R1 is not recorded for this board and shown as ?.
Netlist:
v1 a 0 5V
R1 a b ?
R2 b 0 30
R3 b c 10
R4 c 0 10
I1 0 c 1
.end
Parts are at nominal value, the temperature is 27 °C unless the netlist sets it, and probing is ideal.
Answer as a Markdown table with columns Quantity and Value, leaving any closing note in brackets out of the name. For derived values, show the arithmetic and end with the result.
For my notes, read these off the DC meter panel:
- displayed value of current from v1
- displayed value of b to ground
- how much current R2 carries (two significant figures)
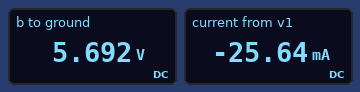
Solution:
| Quantity | Value |
|---|---|
| displayed value of current from v1 | -25.64 mA |
| displayed value of b to ground | 5.692 V |
| how much current R2 carries | (5.692 V) / 30 Ω = 190 mA |
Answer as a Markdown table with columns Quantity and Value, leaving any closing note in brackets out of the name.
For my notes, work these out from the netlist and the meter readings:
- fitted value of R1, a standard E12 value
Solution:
| Quantity | Value |
|---|---|
| fitted value of R1, a standard E12 value | 27 Ω |
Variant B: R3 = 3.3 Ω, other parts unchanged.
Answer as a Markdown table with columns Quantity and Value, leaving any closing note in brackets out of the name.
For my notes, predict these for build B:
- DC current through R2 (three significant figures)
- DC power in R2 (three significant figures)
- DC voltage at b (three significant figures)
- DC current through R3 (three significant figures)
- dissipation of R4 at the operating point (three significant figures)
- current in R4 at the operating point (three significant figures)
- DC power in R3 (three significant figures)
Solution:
| Quantity | Value |
|---|---|
| DC current through R2 | 215 mA |
| DC power in R2 | 1.38 W |
| DC voltage at b | 6.44 V |
| DC current through R3 | 268 mA |
| dissipation of R4 at the operating point | 5.36 W |
| current in R4 at the operating point | 732 mA |
| DC power in R3 | 237 mW |
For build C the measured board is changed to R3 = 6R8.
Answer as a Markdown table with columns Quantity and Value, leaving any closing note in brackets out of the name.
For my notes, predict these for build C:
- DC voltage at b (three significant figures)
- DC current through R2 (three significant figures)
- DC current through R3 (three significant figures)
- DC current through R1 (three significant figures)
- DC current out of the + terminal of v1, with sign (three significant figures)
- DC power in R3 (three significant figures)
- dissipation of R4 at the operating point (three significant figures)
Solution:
| Quantity | Value |
|---|---|
| DC voltage at b | 6.01 V |
| DC current through R2 | 200 mA |
| DC current through R3 | 238 mA |
| DC current through R1 | 37.3 mA |
| DC current out of the + terminal of v1, with sign | -37.3 mA |
| DC power in R3 | 384 mW |
| dissipation of R4 at the operating point | 5.81 W |
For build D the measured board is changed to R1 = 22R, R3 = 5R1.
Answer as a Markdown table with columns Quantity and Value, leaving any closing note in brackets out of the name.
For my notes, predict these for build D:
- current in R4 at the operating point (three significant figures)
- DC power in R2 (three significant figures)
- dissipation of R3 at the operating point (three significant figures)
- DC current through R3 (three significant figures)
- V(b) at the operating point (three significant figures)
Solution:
| Quantity | Value |
|---|---|
| current in R4 at the operating point | 744 mA |
| DC power in R2 | 1.25 W |
| dissipation of R3 at the operating point | 334 mW |
| DC current through R3 | 256 mA |
| V(b) at the operating point | 6.13 V |
